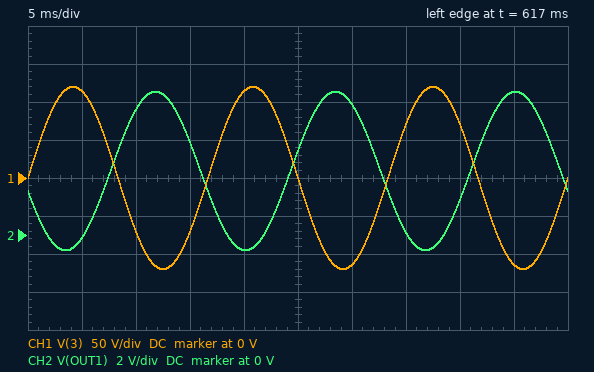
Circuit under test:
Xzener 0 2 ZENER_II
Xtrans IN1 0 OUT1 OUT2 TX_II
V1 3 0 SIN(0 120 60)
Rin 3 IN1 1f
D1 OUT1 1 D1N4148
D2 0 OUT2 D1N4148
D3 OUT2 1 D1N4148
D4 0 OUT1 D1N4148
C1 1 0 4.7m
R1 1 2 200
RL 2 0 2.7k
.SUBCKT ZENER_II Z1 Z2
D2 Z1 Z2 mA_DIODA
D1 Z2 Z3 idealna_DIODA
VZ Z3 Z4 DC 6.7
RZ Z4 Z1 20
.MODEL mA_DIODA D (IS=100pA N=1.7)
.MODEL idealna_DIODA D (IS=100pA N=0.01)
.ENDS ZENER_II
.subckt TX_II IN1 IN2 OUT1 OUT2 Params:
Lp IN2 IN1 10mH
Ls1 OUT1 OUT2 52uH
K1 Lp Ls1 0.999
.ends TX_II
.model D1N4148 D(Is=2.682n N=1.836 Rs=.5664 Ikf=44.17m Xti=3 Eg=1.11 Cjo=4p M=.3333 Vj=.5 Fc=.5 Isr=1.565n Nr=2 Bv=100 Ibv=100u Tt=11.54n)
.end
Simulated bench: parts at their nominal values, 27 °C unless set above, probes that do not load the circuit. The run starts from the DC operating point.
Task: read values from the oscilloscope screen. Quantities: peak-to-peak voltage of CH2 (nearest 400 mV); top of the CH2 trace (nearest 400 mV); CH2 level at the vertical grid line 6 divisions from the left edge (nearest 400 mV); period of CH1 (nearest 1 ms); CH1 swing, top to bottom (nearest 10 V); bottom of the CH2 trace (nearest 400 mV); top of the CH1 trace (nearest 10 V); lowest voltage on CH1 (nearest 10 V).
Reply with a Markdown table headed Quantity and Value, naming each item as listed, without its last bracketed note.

| Quantity | Value |
|---|---|
| peak-to-peak voltage of CH2 | 8.4 V |
| top of the CH2 trace | 7.6 V |
| CH2 level at the vertical grid line 6 divisions from the left edge | 6.8 V |
| period of CH1 | 17 ms |
| CH1 swing, top to bottom | 240 V |
| bottom of the CH2 trace | -800 mV |
| top of the CH1 trace | 120 V |
| lowest voltage on CH1 | -120 V |
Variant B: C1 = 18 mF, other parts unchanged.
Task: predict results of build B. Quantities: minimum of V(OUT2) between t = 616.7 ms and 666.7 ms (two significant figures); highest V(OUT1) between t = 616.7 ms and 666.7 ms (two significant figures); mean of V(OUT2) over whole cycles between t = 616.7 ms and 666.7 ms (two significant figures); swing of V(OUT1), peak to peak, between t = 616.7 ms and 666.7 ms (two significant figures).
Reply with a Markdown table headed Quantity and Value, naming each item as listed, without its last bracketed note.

| Quantity | Value |
|---|---|
| minimum of V(OUT2) between t = 616.7 ms and 666.7 ms | -940 mV |
| highest V(OUT1) between t = 616.7 ms and 666.7 ms | 7.4 V |
| mean of V(OUT2) over whole cycles between t = 616.7 ms and 666.7 ms | 3.2 V |
| swing of V(OUT1), peak to peak, between t = 616.7 ms and 666.7 ms | 8.4 V |
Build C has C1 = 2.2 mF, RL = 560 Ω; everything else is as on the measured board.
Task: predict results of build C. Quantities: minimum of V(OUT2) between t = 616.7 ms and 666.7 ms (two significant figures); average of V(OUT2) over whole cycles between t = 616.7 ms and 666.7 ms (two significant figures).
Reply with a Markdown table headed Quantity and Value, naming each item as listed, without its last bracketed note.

| Quantity | Value |
|---|---|
| minimum of V(OUT2) between t = 616.7 ms and 666.7 ms | -910 mV |
| average of V(OUT2) over whole cycles between t = 616.7 ms and 666.7 ms | 3.3 V |
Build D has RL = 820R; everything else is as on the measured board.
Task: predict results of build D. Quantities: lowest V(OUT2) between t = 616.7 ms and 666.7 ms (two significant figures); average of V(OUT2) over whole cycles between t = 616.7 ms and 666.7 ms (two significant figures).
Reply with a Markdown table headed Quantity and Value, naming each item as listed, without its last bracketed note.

| Quantity | Value |
|---|---|
| lowest V(OUT2) between t = 616.7 ms and 666.7 ms | -880 mV |
| average of V(OUT2) over whole cycles between t = 616.7 ms and 666.7 ms | 3.3 V |
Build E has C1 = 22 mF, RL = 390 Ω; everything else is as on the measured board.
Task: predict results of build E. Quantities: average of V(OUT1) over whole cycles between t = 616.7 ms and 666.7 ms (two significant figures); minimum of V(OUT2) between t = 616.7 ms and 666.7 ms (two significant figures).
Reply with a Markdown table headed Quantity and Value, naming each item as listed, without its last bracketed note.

| Quantity | Value |
|---|---|
| average of V(OUT1) over whole cycles between t = 616.7 ms and 666.7 ms | 3.2 V |
| minimum of V(OUT2) between t = 616.7 ms and 666.7 ms | -1.0 V |
